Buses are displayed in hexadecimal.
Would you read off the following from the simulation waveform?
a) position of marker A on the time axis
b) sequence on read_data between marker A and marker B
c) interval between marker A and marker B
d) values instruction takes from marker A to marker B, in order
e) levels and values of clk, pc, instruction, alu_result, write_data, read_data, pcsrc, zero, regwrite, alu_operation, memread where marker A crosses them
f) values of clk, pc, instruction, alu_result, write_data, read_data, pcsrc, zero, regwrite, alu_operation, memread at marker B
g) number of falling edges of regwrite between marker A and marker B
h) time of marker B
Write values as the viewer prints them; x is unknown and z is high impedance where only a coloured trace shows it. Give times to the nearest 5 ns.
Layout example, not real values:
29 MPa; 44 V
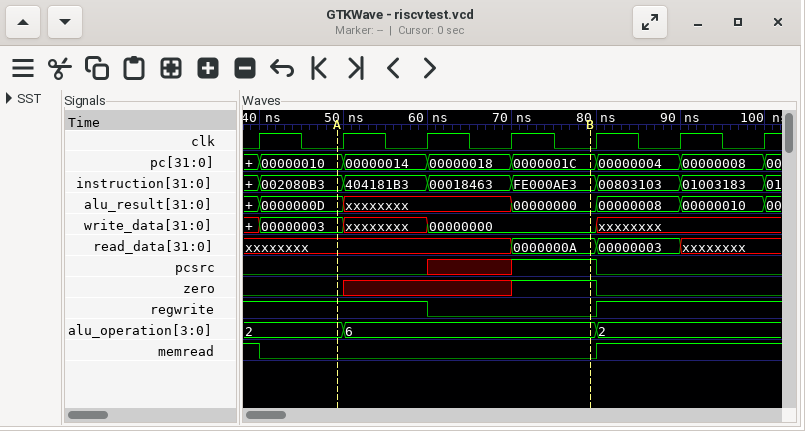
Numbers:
50 ns; xxxxxxxx, 0000000A; 30 ns; 002080B3, 404181B3, 00018463, FE000AE3; clk=0, pc=00000010, instruction=002080B3, alu_result=0000000D, write_data=00000003, read_data=xxxxxxxx, pcsrc=0, zero=0, regwrite=1, alu_operation=2, memread=0; clk=0, pc=0000001C, instruction=FE000AE3, alu_result=00000000, write_data=00000000, read_data=0000000A, pcsrc=1, zero=1, regwrite=0, alu_operation=6, memread=0; 1; 80 ns
